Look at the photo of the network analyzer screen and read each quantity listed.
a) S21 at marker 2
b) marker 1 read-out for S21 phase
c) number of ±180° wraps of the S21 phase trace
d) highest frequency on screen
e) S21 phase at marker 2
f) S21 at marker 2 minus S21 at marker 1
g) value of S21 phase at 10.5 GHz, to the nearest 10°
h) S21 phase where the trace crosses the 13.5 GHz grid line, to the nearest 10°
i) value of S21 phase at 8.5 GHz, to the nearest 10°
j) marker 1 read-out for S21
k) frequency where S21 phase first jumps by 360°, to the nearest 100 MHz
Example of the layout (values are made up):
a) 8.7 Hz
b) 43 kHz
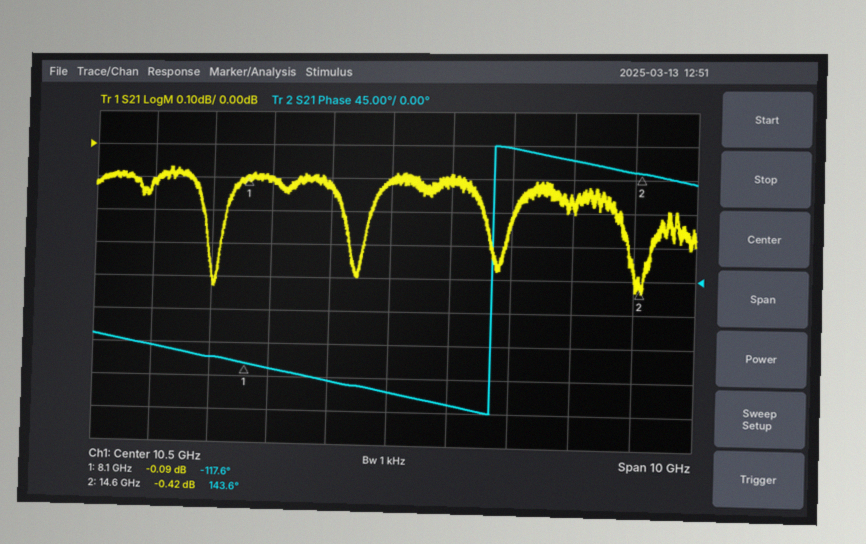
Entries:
a) -0.42 dB
b) -117.6°
c) 1
d) 15.5 GHz
e) 143.6°
f) -0.33 dB
g) -150°
h) 160°
i) -120°
j) -0.09 dB
k) 12.2 GHz
